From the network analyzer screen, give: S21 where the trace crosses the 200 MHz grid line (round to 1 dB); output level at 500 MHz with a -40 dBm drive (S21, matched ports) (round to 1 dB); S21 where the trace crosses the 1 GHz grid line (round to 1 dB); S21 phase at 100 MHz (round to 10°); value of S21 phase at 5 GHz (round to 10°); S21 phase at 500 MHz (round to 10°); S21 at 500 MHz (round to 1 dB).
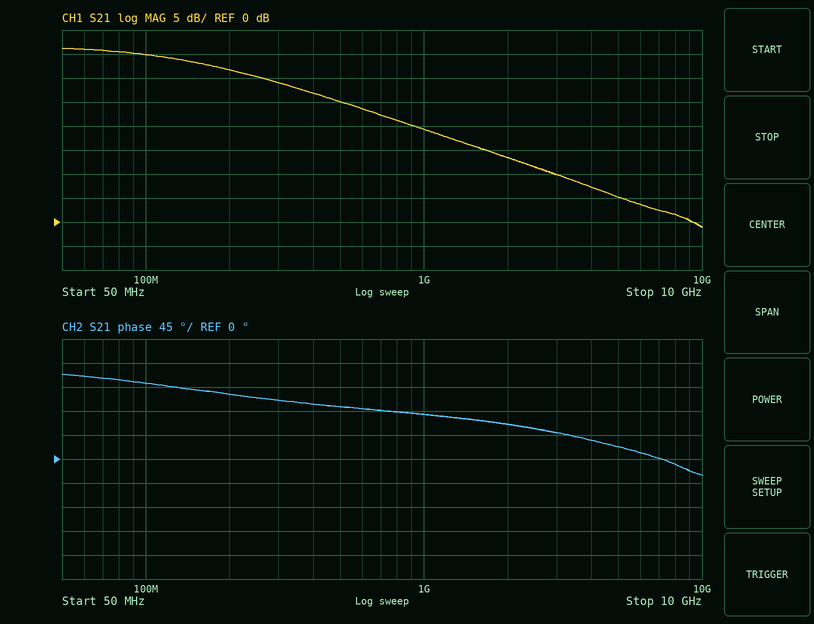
32 dB
-15 dBm
19 dB
140°
20°
100°
25 dB
